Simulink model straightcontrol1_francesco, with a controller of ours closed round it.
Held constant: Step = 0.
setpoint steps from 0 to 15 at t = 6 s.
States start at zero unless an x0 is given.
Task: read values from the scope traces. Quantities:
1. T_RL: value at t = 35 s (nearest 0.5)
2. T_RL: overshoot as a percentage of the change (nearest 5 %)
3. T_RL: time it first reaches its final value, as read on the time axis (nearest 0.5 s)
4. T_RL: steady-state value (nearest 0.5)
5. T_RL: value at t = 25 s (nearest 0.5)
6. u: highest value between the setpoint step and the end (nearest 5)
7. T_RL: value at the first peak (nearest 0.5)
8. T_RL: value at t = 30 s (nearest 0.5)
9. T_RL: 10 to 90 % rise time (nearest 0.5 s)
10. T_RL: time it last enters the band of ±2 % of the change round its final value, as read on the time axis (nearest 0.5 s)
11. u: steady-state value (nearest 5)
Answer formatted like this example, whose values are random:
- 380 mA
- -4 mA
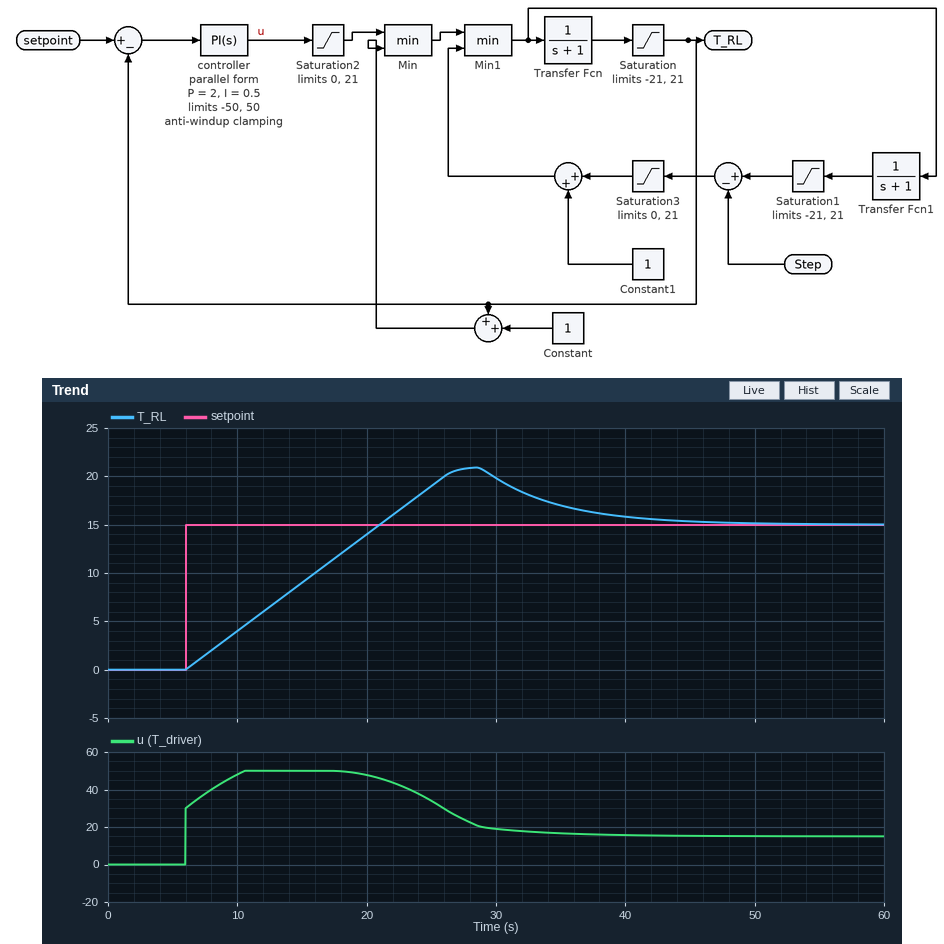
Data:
- 17.0
- 40 %
- 21.0 s
- 15.0
- 19.0
- 50
- 21.0
- 20.0
- 12.0 s
- 45.5 s
- 15
